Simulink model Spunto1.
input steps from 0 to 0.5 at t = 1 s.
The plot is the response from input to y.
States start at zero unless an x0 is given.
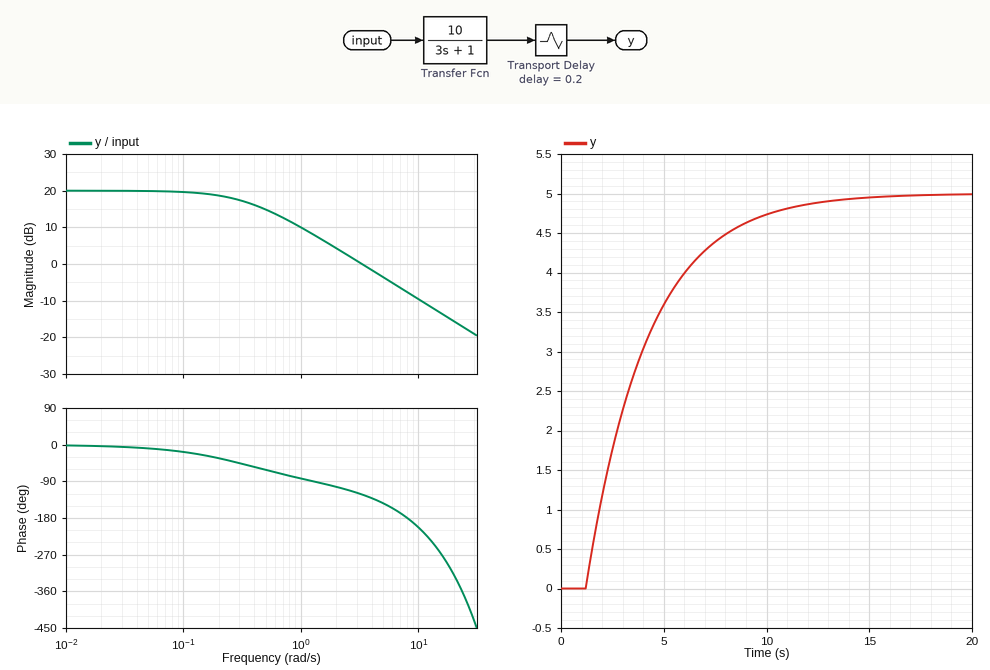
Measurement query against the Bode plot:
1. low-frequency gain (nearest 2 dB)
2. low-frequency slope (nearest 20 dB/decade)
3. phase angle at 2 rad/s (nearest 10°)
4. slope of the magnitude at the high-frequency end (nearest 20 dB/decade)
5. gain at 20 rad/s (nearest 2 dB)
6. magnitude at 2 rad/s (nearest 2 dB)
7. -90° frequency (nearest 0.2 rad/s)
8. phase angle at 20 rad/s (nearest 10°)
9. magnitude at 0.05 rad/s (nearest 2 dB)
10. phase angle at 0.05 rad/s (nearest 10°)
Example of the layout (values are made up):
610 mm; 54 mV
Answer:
20 dB; 0 dB/decade; -100°; -20 dB/decade; -16 dB; 4 dB; 1.2 rad/s; -320°; 20 dB; -10°
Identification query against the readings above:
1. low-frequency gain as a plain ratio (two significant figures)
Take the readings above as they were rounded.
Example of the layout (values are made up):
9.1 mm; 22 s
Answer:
10
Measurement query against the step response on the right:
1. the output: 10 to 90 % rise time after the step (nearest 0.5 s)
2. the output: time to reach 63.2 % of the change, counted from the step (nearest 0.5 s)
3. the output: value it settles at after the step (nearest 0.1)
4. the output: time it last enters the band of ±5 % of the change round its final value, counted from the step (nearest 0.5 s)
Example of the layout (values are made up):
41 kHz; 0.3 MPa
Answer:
6.5 s; 3.0 s; 5.0; 9.0 s
